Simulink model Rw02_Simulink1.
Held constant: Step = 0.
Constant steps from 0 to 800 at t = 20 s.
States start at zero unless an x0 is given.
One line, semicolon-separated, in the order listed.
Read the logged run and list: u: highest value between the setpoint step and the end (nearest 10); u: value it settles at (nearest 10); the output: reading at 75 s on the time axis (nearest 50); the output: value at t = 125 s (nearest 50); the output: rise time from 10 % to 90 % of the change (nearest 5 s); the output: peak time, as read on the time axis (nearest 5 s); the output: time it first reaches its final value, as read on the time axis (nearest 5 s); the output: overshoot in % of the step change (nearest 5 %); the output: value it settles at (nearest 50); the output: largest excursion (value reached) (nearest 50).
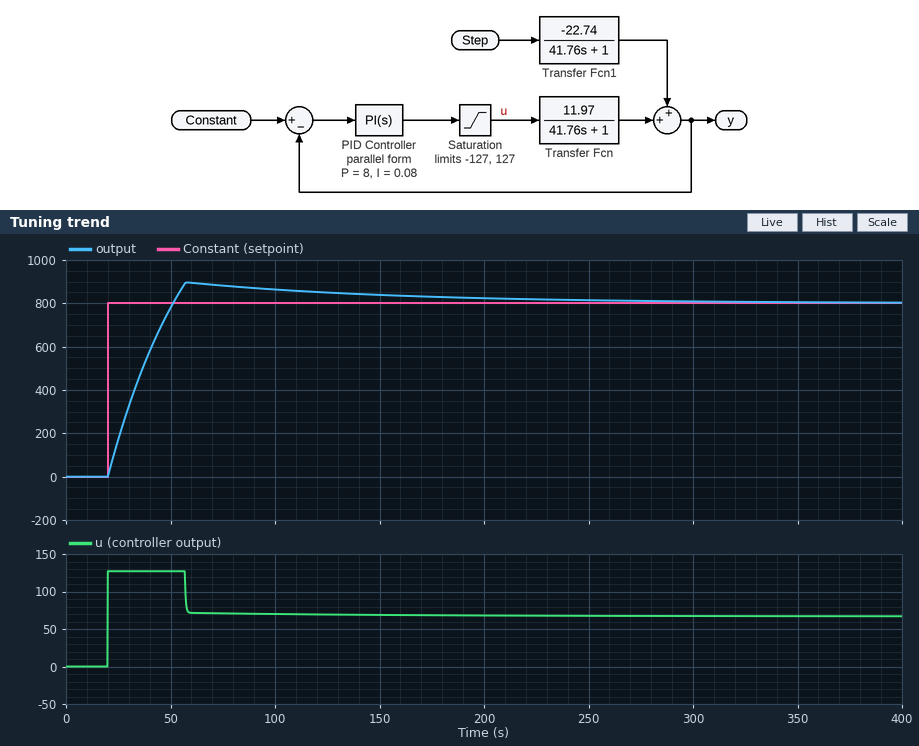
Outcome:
130; 70; 900; 850; 25 s; 60 s; 50 s; 10 %; 800; 900
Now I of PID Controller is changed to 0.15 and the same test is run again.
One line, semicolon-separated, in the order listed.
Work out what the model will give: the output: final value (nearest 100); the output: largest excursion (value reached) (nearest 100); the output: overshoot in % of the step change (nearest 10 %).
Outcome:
800; 1000; 20 %
